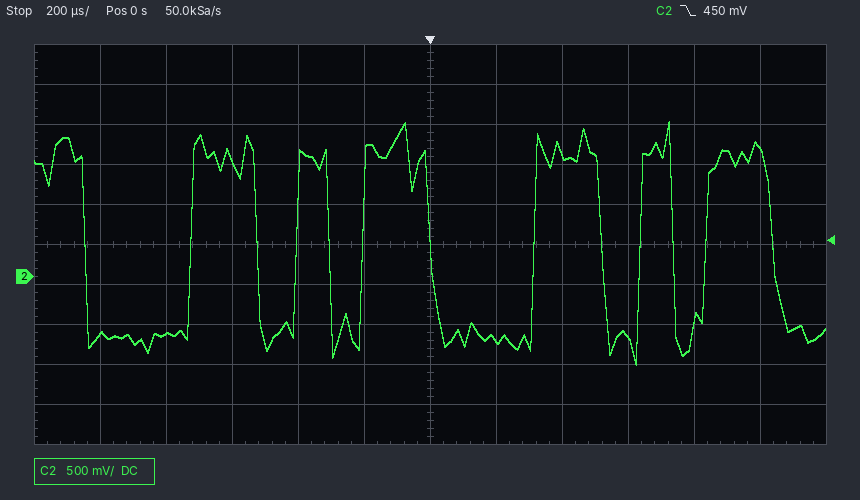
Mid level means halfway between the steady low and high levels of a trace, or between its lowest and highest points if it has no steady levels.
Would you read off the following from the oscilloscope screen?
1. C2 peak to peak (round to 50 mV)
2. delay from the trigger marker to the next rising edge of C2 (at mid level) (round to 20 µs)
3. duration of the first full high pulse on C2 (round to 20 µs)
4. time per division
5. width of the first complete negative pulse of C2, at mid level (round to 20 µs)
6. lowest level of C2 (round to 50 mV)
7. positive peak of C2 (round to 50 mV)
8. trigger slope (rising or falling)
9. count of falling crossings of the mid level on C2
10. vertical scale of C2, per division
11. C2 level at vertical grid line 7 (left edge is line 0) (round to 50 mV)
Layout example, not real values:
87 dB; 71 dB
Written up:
3.05 V; 320 µs; 200 µs; 200 µs; 320 µs; -1.10 V; 1.95 V; falling; 7; 500 mV; -800 mV
